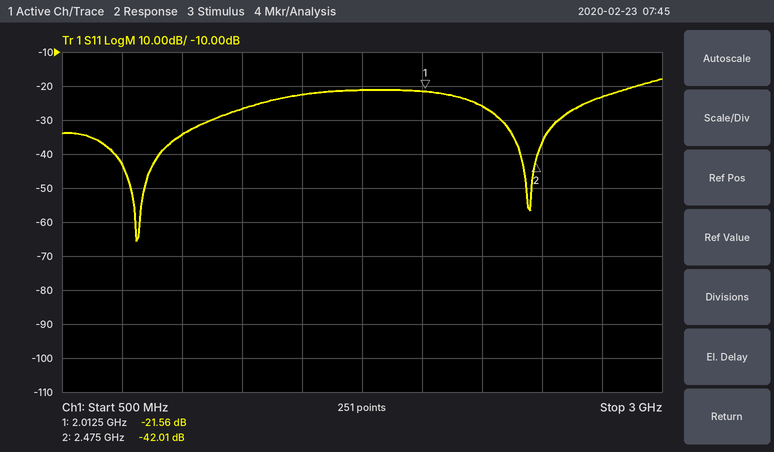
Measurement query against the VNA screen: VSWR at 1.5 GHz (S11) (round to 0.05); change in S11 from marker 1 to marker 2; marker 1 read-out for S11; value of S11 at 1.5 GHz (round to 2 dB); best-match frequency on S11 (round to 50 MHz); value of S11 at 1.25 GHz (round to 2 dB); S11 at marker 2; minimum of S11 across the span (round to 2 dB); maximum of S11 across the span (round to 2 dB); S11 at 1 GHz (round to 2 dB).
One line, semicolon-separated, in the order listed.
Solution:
1.15; -20.45 dB; -21.56 dB; -22 dB; 800 MHz; -26 dB; -42.01 dB; -66 dB; -18 dB; -34 dB
